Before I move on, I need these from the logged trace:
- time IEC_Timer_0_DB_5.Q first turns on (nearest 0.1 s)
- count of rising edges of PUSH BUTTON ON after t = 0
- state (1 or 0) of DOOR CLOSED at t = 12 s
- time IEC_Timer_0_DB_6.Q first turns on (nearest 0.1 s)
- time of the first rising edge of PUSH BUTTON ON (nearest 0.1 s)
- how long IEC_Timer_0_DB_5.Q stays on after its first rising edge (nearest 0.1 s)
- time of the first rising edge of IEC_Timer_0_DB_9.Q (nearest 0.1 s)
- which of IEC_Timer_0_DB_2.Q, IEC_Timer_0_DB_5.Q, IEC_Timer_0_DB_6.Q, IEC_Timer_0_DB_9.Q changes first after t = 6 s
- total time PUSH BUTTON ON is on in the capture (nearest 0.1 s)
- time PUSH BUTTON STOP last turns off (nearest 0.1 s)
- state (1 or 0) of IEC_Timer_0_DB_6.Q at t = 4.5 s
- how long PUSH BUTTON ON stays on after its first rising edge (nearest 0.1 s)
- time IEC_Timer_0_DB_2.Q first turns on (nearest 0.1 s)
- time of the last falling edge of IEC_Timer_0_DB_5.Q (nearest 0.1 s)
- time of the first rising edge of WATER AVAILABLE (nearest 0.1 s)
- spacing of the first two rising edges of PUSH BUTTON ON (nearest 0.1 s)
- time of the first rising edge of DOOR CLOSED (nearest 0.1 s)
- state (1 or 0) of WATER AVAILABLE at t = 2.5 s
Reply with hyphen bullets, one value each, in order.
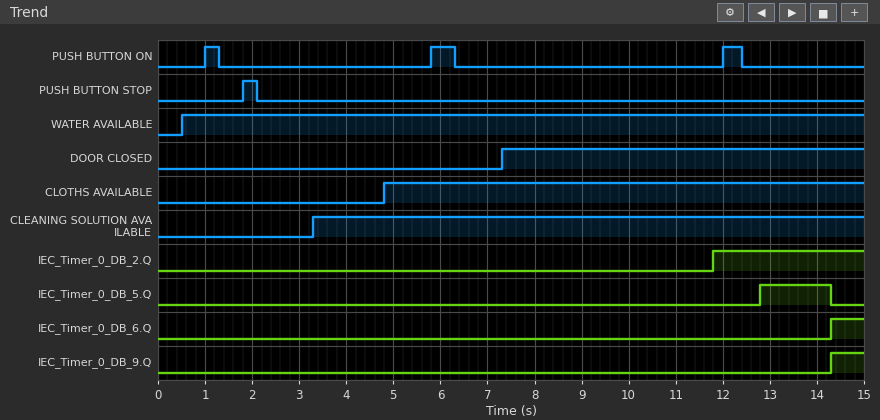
- 12.8 s
- 3
- 1
- 14.3 s
- 1.0 s
- 1.5 s
- 14.3 s
- IEC_Timer_0_DB_2.Q
- 1.2 s
- 2.1 s
- 0
- 0.3 s
- 11.8 s
- 14.3 s
- 0.5 s
- 4.8 s
- 7.3 s
- 1
